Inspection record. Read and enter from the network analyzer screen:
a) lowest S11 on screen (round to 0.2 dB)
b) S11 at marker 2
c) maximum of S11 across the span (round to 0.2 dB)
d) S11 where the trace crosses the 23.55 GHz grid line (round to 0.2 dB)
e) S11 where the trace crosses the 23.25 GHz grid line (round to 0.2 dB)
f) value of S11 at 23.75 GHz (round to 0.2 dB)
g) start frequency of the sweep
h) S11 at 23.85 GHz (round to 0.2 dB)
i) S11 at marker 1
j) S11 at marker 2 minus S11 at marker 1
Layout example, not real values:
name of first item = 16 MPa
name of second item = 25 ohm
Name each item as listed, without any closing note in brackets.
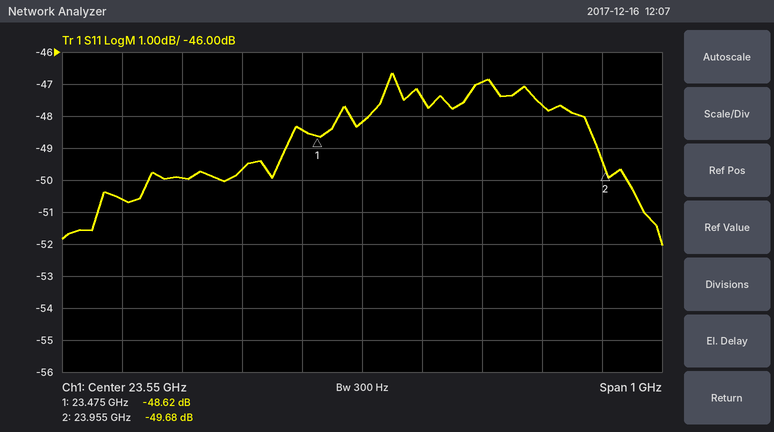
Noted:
lowest S11 on screen = -52.0 dB
S11 at marker 2 = -49.68 dB
maximum of S11 across the span = -46.6 dB
S11 where the trace crosses the 23.55 GHz grid line = -48.2 dB
S11 where the trace crosses the 23.25 GHz grid line = -50.0 dB
value of S11 at 23.75 GHz = -47.0 dB
start frequency of the sweep = 23.05 GHz
S11 at 23.85 GHz = -47.6 dB
S11 at marker 1 = -48.62 dB
S11 at marker 2 minus S11 at marker 1 = -1.06 dB
